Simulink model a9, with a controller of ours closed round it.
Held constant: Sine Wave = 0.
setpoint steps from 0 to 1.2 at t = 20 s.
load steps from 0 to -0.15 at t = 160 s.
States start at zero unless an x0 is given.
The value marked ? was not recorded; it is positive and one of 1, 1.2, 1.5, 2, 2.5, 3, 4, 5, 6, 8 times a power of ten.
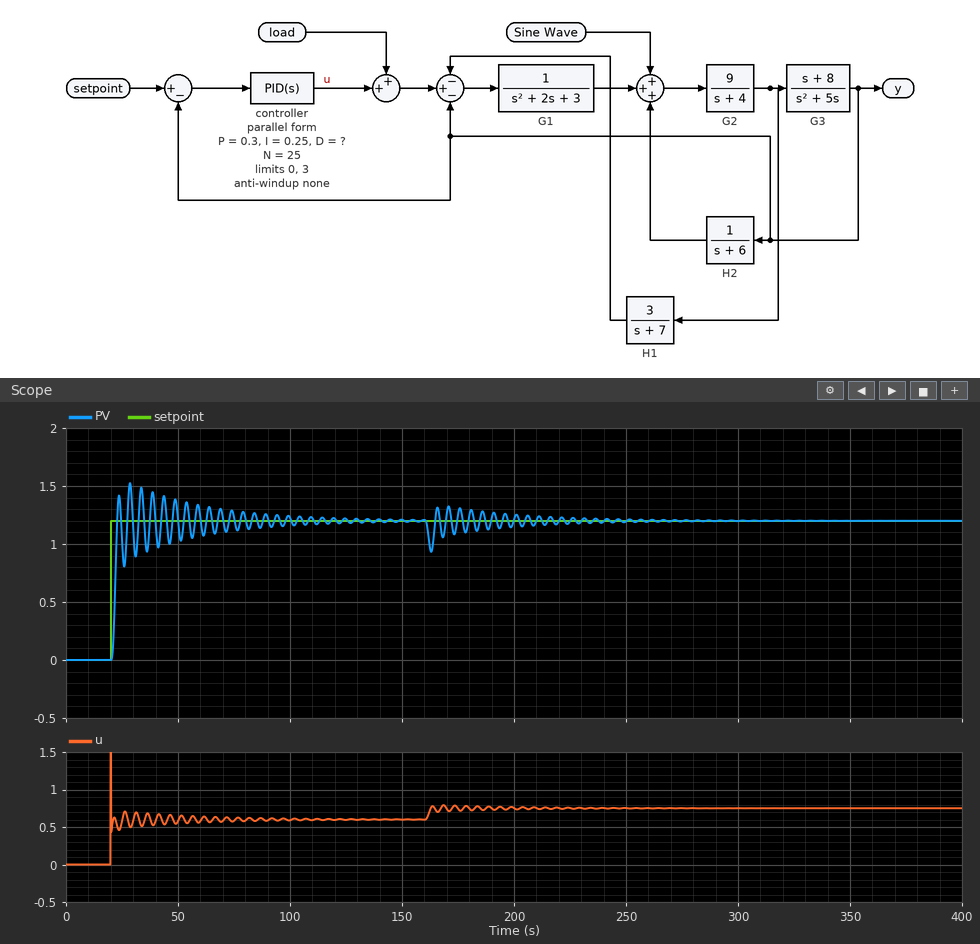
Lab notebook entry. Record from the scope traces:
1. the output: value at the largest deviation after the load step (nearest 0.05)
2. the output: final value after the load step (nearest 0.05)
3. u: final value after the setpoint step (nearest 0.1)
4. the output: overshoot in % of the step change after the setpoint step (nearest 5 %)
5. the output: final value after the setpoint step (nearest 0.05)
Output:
0.95
1.20
0.6
25 %
1.20
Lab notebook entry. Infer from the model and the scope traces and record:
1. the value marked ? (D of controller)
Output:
0.08
